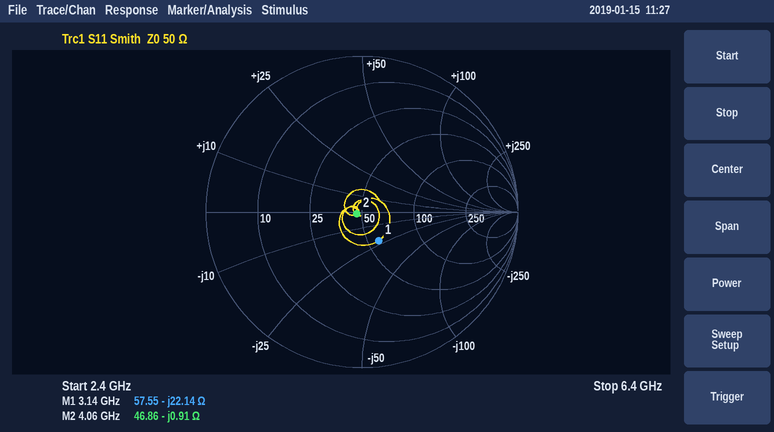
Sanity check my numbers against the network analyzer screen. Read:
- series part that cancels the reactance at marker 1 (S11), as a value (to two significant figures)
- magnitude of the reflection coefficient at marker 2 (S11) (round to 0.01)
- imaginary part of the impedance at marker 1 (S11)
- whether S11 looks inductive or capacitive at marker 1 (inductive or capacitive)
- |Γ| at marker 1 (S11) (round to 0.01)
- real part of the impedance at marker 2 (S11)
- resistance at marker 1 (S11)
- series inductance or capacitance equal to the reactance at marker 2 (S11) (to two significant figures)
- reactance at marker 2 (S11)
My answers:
1.1 nH
0.03
-22.14 Ω
capacitive
0.21
46.86 Ω
57.55 Ω
43 pF
-0.91 Ω
